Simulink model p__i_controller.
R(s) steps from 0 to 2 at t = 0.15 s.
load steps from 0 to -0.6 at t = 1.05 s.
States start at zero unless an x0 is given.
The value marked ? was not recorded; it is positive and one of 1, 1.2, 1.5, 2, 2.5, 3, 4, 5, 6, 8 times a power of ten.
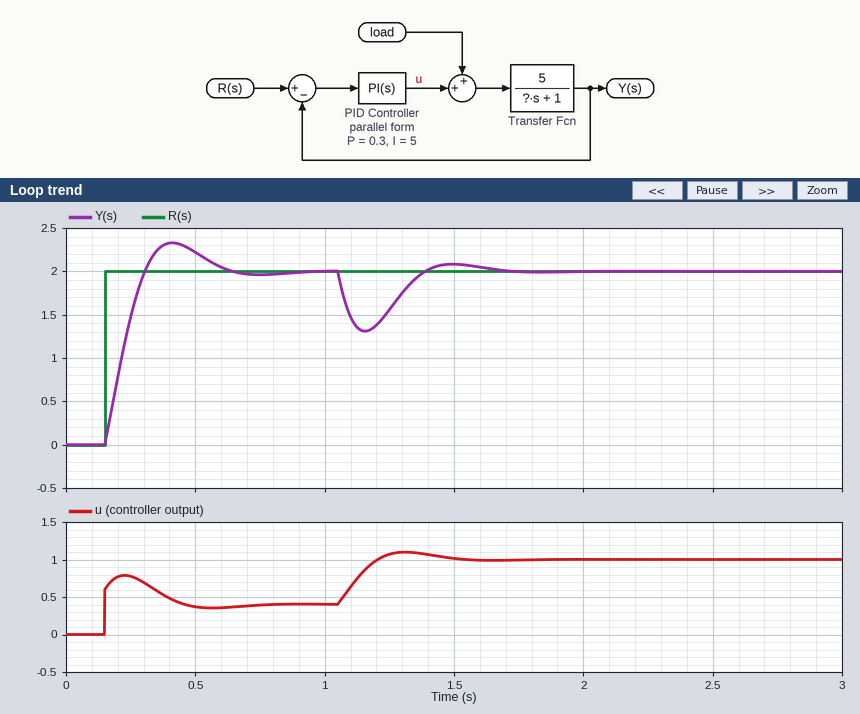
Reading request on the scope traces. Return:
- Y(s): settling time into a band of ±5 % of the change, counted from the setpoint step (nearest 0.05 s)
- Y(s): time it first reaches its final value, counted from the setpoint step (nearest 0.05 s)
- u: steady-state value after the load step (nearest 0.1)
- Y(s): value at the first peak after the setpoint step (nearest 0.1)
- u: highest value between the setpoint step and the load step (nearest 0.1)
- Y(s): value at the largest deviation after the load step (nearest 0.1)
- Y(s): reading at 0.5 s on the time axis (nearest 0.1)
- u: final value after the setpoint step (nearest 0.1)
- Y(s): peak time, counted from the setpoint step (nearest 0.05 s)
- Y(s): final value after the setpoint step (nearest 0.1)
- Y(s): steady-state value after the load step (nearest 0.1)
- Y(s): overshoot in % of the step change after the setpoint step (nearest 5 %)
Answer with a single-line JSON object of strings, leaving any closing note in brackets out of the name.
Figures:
{"Y(s): settling time into a band of ±5 % of the change, counted from the setpoint step": "0.40 s", "Y(s): time it first reaches its final value, counted from the setpoint step": "0.15 s", "u: steady-state value after the load step": "1.0", "Y(s): value at the first peak after the setpoint step": "2.3", "u: highest value between the setpoint step and the load step": "0.8", "Y(s): value at the largest deviation after the load step": "1.3", "Y(s): reading at 0.5 s on the time axis": "2.2", "u: final value after the setpoint step": "0.4", "Y(s): peak time, counted from the setpoint step": "0.25 s", "Y(s): final value after the setpoint step": "2.0", "Y(s): steady-state value after the load step": "2.0", "Y(s): overshoot in % of the step change after the setpoint step": "15 %"}
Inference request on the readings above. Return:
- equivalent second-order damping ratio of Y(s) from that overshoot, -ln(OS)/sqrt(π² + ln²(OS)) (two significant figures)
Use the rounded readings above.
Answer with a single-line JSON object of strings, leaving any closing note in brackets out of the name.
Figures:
{"equivalent second-order damping ratio of Y(s) from that overshoot, -ln(OS)/sqrt(π² + ln²(OS))": "0.52"}
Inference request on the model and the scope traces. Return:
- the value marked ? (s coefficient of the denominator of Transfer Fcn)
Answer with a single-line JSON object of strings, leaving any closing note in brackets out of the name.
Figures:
{"the value marked ?": "0.2"}
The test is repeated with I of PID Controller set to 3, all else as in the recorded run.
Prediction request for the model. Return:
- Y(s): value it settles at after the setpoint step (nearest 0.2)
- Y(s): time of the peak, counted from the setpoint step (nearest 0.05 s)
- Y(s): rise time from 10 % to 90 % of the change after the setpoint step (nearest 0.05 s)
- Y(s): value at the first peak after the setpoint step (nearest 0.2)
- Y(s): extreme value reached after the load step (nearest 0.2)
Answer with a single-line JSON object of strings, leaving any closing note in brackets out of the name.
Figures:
{"Y(s): value it settles at after the setpoint step": "2.0", "Y(s): time of the peak, counted from the setpoint step": "0.35 s", "Y(s): rise time from 10 % to 90 % of the change after the setpoint step": "0.15 s", "Y(s): value at the first peak after the setpoint step": "2.2", "Y(s): extreme value reached after the load step": "1.2"}
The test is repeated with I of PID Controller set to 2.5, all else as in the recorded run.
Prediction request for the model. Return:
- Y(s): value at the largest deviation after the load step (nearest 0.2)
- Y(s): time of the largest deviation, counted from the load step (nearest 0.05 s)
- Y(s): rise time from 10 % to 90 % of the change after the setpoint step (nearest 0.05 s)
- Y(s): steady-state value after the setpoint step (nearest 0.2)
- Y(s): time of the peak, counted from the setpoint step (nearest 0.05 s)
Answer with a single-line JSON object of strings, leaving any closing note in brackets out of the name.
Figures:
{"Y(s): value at the largest deviation after the load step": "1.2", "Y(s): time of the largest deviation, counted from the load step": "0.15 s", "Y(s): rise time from 10 % to 90 % of the change after the setpoint step": "0.20 s", "Y(s): steady-state value after the setpoint step": "2.0", "Y(s): time of the peak, counted from the setpoint step": "0.40 s"}
